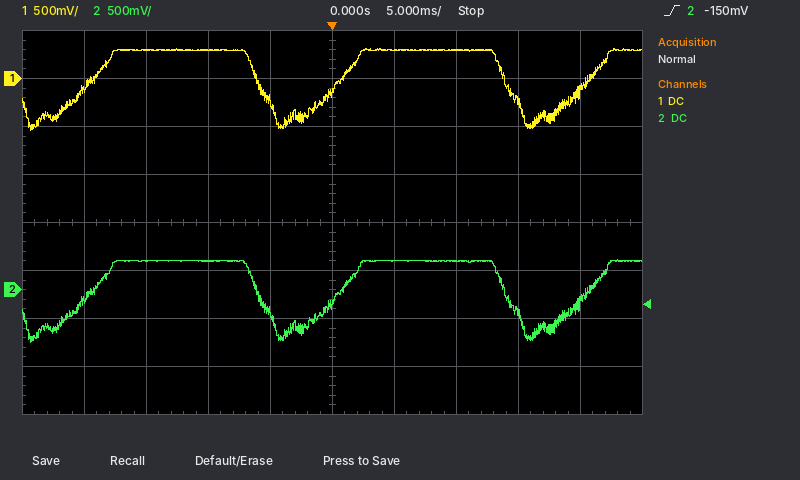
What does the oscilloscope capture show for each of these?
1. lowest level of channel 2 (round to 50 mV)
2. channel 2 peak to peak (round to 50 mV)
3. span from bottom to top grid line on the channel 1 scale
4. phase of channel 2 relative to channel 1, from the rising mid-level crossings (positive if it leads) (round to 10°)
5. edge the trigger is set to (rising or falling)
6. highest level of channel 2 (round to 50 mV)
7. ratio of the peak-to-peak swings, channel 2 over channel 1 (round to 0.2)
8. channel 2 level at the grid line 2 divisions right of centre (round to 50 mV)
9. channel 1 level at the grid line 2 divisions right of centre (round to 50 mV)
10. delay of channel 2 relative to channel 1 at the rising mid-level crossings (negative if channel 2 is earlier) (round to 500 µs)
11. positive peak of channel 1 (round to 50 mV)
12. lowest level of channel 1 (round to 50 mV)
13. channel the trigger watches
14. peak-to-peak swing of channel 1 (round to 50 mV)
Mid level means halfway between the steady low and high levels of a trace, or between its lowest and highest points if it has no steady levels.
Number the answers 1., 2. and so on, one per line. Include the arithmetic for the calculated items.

1. -550 mV
2. 300 mV − (-550 mV) = 850 mV
3. 4 V
4. 0°
5. rising
6. 300 mV
7. 850 mV / 850 mV ≈ 1.0
8. 300 mV
9. 300 mV
10. 0.0 ms
11. 300 mV
12. -550 mV
13. channel 2
14. 300 mV − (-550 mV) = 850 mV
